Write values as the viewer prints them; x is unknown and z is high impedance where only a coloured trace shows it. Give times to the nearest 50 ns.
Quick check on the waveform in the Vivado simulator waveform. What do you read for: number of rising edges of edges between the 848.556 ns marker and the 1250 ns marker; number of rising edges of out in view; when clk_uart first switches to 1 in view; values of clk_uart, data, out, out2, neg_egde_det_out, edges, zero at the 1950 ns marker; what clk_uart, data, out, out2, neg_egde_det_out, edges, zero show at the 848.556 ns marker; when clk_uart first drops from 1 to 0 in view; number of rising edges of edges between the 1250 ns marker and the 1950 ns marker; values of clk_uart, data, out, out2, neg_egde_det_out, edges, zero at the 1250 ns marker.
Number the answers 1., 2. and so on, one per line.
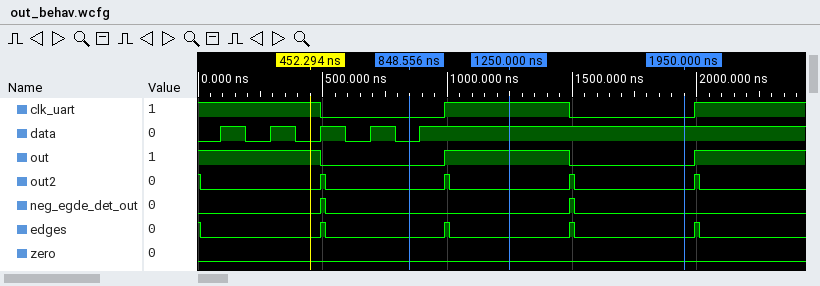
1. 1
2. 2
3. 1000 ns
4. clk_uart=0, data=1, out=0, out2=0, neg_egde_det_out=0, edges=0, zero=0
5. clk_uart=0, data=0, out=0, out2=0, neg_egde_det_out=0, edges=0, zero=0
6. 500 ns
7. 1
8. clk_uart=1, data=1, out=1, out2=0, neg_egde_det_out=0, edges=0, zero=0
